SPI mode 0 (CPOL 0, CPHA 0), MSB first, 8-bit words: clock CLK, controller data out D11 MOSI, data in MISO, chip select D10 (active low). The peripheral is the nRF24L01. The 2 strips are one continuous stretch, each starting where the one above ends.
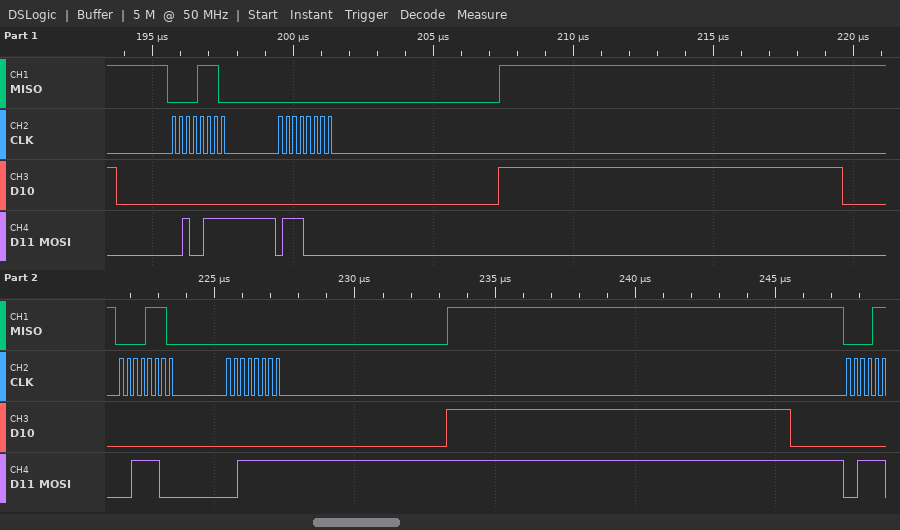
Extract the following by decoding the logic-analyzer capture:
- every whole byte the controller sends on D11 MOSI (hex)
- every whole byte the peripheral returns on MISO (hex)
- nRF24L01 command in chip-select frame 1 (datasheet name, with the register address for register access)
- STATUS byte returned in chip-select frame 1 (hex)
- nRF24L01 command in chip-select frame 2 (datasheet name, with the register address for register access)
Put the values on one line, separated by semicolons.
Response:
27 70 3C 3F; 0E 00 0E 00; W_REGISTER 0x07; 0x0E; W_REGISTER 0x1C
